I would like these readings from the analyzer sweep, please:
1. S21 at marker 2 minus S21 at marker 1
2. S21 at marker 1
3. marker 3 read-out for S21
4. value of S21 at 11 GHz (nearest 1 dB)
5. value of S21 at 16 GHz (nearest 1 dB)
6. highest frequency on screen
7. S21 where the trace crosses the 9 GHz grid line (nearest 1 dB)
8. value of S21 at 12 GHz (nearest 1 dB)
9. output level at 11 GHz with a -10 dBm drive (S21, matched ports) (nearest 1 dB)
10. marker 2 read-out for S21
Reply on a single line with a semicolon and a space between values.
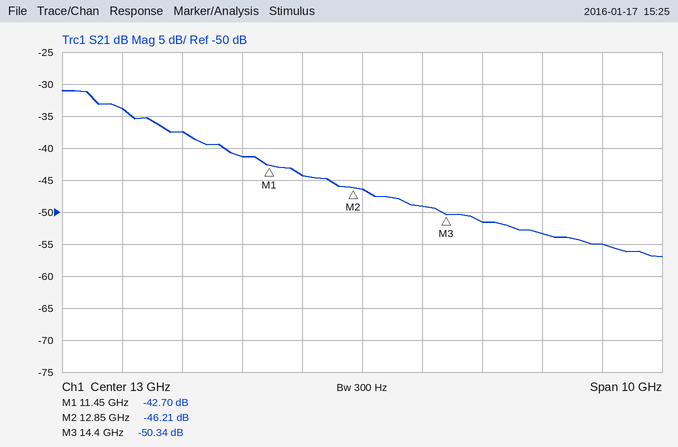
-3.51 dB; -42.70 dB; -50.34 dB; -41 dB; -53 dB; 18 GHz; -34 dB; -44 dB; -51 dBm; -46.21 dB
